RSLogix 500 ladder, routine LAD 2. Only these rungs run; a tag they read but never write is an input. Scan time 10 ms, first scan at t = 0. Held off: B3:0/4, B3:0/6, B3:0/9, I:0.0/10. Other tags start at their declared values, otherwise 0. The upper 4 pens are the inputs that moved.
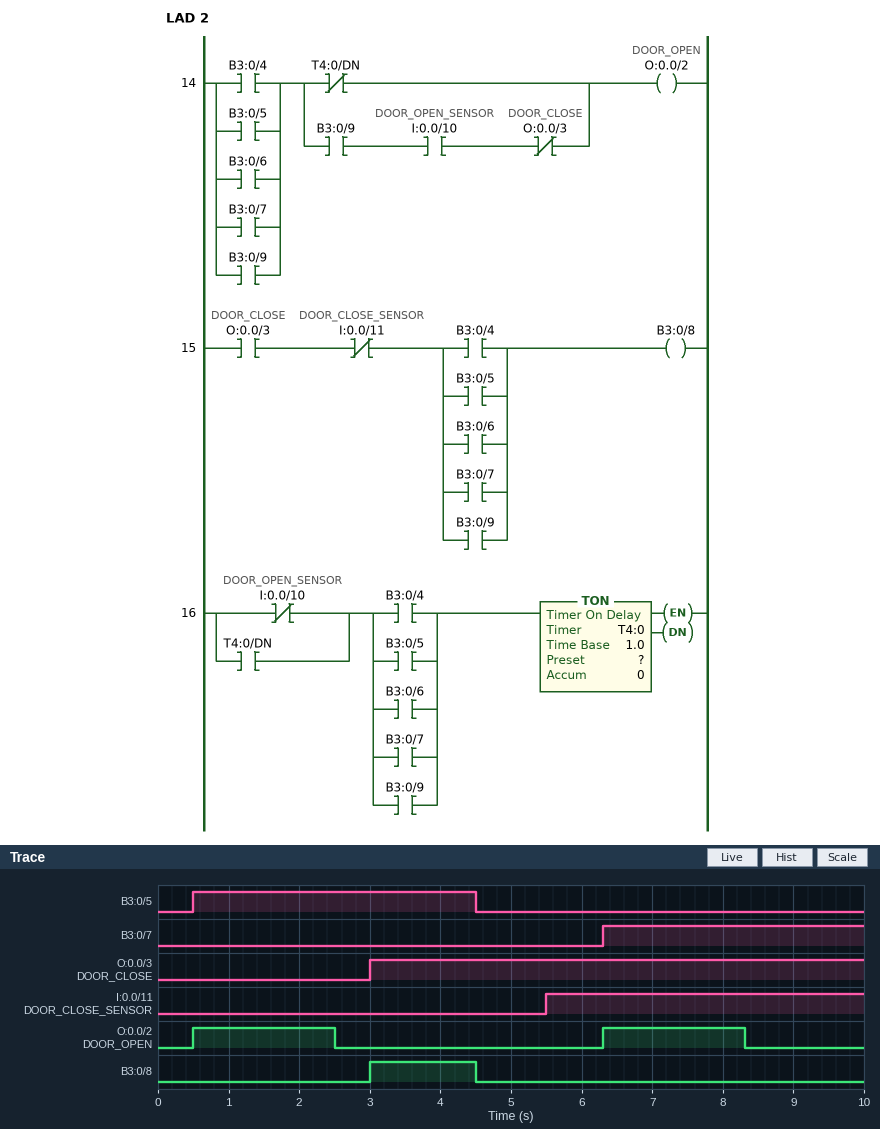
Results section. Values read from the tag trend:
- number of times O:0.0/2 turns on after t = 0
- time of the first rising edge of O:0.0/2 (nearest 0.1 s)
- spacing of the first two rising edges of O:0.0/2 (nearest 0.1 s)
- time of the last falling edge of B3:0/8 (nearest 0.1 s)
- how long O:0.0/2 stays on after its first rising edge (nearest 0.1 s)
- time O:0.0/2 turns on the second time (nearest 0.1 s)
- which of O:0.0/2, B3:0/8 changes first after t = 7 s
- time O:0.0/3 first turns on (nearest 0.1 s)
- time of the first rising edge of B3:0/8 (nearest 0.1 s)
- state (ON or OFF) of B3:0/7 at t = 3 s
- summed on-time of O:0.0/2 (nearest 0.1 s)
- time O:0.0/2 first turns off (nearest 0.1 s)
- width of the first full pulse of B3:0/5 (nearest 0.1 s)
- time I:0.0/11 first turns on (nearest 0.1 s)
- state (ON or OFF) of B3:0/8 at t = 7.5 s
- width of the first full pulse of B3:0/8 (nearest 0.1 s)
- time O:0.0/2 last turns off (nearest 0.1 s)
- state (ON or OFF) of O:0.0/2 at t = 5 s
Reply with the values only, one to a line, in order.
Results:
2
0.5 s
5.8 s
4.5 s
2.0 s
6.3 s
O:0.0/2
3.0 s
3.0 s
OFF
4.0 s
2.5 s
4.0 s
5.5 s
OFF
1.5 s
8.3 s
OFF
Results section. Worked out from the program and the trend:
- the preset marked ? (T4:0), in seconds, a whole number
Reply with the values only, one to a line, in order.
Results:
2 s
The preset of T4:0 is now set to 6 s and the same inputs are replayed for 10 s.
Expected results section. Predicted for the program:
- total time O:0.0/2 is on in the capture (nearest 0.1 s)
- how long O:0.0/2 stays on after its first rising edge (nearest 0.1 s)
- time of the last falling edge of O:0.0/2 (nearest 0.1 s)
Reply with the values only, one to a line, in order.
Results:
7.7 s
4.0 s
4.5 s
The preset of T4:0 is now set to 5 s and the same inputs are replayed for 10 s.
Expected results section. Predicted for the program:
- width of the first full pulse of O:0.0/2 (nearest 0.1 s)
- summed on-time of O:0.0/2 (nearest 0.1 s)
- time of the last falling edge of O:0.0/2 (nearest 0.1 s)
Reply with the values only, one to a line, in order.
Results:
4.0 s
7.7 s
4.5 s
